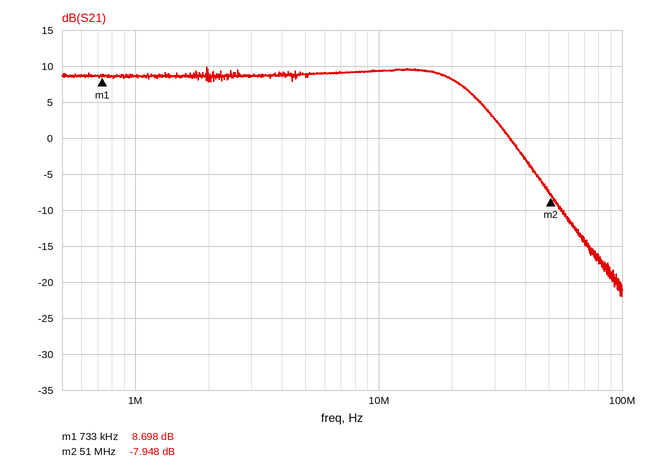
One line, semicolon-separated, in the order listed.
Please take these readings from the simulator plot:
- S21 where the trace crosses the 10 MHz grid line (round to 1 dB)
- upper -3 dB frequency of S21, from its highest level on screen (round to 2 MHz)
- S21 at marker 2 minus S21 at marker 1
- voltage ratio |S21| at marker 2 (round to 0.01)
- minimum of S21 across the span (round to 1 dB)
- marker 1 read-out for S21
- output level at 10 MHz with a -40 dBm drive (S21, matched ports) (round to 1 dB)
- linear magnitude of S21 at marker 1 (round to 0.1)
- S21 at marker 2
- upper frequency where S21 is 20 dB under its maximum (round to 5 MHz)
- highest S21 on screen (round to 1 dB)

9 dB; 22 MHz; -16.646 dB; 0.40; -22 dB; 8.698 dB; -31 dBm; 2.7; -7.948 dB; 55 MHz; 10 dB
